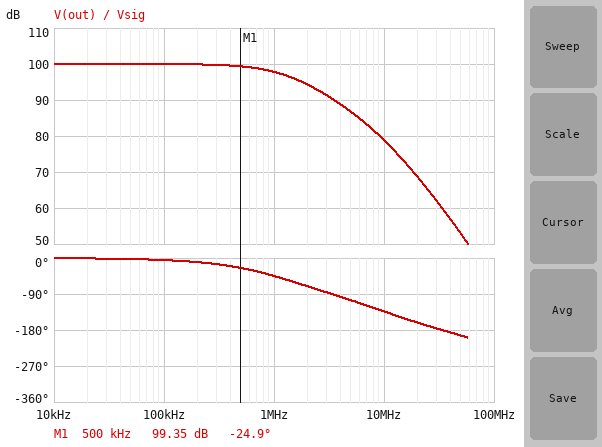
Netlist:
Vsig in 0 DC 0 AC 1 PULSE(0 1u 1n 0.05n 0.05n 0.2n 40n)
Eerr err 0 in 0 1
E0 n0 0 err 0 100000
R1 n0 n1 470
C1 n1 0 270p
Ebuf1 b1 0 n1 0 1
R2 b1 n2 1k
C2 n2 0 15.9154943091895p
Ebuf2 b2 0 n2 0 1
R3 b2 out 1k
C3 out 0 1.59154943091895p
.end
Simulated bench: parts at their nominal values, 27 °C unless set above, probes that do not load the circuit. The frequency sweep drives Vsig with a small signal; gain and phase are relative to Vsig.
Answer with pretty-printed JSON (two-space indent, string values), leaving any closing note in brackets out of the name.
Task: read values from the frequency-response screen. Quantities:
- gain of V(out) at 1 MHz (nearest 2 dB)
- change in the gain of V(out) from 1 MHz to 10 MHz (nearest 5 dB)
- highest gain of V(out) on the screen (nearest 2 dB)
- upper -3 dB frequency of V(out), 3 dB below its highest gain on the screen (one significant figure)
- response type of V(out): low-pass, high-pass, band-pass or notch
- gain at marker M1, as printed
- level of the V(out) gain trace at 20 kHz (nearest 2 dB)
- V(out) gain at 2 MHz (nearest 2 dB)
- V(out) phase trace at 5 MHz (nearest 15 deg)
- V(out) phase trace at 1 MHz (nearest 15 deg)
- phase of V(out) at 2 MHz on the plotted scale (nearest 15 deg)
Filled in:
{
  "gain of V(out) at 1 MHz": "98 dB",
  "change in the gain of V(out) from 1 MHz to 10 MHz": "-20 dB",
  "highest gain of V(out) on the screen": "100 dB",
  "upper -3 dB frequency of V(out), 3 dB below its highest gain on the screen": "1 MHz",
  "response type of V(out): low-pass, high-pass, band-pass or notch": "low-pass",
  "gain at marker M1, as printed": "99.35 dB",
  "level of the V(out) gain trace at 20 kHz": "100 dB",
  "V(out) gain at 2 MHz": "94 dB",
  "V(out) phase trace at 5 MHz": "-105 deg",
  "V(out) phase trace at 1 MHz": "-45 deg",
  "phase of V(out) at 2 MHz on the plotted scale": "-75 deg"
}
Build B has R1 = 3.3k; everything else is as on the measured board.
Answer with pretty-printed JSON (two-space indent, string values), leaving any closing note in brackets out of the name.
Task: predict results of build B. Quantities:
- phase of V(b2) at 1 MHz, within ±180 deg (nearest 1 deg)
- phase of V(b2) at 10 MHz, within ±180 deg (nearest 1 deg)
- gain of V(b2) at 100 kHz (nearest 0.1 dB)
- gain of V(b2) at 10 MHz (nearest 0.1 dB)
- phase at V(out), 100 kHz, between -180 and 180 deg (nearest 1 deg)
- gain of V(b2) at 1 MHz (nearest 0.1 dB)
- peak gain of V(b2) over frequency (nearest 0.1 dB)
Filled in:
{
  "phase of V(b2) at 1 MHz, within ±180 deg": "-86 deg",
  "phase of V(b2) at 10 MHz, within ±180 deg": "-134 deg",
  "gain of V(b2) at 100 kHz": "98.8 dB",
  "gain of V(b2) at 10 MHz": "62.0 dB",
  "phase at V(out), 100 kHz, between -180 and 180 deg": "-30 deg",
  "gain of V(b2) at 1 MHz": "84.9 dB",
  "peak gain of V(b2) over frequency": "100.0 dB"
}
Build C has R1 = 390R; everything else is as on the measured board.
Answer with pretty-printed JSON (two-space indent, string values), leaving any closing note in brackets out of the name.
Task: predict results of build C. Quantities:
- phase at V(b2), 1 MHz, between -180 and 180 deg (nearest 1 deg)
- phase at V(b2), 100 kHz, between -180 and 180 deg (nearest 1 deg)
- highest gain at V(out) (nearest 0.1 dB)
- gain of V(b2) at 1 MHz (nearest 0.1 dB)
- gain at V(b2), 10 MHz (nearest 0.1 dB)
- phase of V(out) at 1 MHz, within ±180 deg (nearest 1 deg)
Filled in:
{
  "phase at V(b2), 1 MHz, between -180 and 180 deg": "-39 deg",
  "phase at V(b2), 100 kHz, between -180 and 180 deg": "-4 deg",
  "highest gain at V(out)": "100.0 dB",
  "gain of V(b2) at 1 MHz": "98.4 dB",
  "gain at V(b2), 10 MHz": "80.5 dB",
  "phase of V(out) at 1 MHz, within ±180 deg": "-40 deg"
}
